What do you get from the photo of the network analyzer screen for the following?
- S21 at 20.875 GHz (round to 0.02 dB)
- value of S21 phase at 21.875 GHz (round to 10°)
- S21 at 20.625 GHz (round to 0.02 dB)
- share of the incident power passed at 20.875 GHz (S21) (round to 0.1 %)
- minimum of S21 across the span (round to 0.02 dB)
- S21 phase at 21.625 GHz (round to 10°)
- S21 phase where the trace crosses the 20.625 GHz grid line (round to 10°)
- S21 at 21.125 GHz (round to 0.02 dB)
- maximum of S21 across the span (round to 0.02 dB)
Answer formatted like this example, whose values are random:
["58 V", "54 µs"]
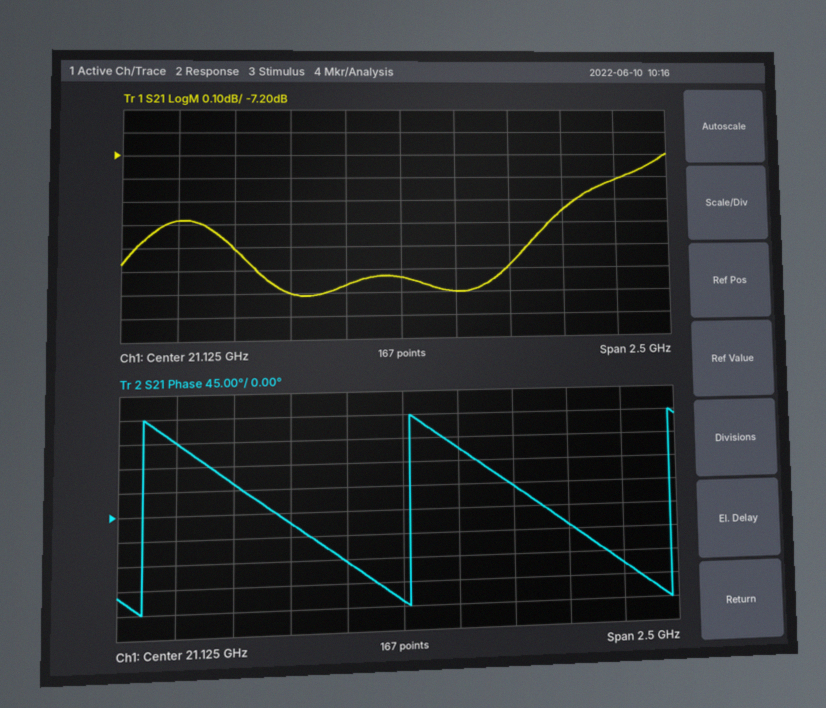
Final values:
["-7.76 dB", "-40°", "-7.80 dB", "16.7 %", "-7.82 dB", "40°", "-20°", "-7.74 dB", "-7.20 dB"]
